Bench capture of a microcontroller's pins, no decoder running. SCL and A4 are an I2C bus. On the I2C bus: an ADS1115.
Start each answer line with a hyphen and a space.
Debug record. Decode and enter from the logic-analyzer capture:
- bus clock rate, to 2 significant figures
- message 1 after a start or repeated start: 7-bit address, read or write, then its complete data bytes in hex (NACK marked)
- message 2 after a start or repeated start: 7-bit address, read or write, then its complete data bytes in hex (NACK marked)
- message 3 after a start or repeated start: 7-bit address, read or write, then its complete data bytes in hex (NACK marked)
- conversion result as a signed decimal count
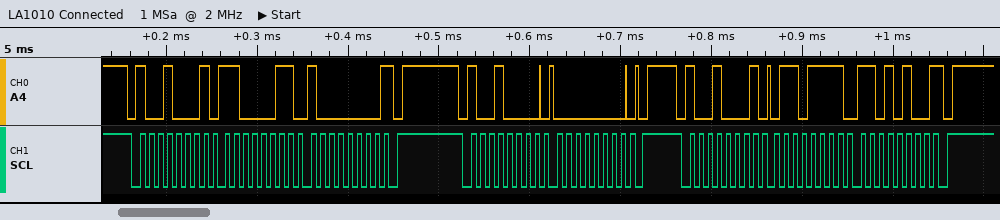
- 100 kHz
- 0x48 read: C3 80 NACK
- 0x48 write: 00
- 0x48 read: 6F D4 NACK
- 28628
